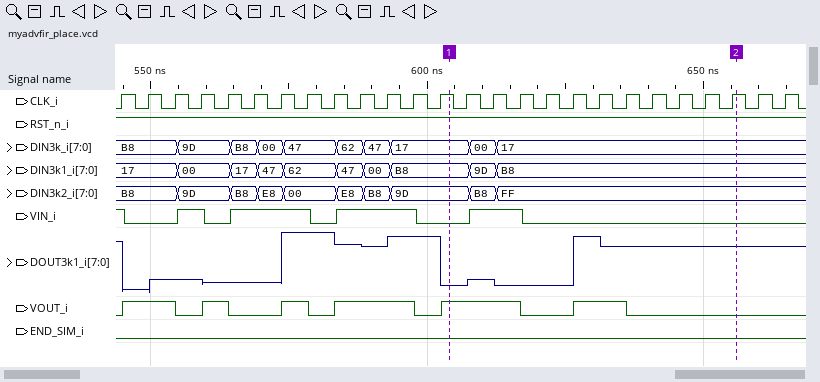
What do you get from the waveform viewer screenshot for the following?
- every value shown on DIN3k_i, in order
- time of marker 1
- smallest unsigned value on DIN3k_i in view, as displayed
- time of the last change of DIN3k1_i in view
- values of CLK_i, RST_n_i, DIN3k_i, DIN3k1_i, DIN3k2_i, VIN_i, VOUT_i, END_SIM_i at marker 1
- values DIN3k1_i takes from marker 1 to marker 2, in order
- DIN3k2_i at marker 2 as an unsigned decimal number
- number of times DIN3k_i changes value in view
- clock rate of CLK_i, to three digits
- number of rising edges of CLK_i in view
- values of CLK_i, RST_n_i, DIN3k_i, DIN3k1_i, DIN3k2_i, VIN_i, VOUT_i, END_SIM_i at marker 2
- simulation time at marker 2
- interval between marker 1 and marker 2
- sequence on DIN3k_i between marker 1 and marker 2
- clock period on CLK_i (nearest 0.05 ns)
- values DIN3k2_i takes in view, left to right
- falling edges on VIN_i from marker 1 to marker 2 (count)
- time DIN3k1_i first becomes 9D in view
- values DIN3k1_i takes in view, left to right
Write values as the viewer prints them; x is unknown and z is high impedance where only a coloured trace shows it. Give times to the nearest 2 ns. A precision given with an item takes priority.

B8, 9D, B8, 00, 47, 62, 47, 17, 00, 17
604 ns
00
612 ns
CLK_i=1, RST_n_i=1, DIN3k_i=17, DIN3k1_i=B8, DIN3k2_i=9D, VIN_i=0, VOUT_i=1, END_SIM_i=0
B8, 9D, B8
255
9
208 MHz
26
CLK_i=1, RST_n_i=1, DIN3k_i=17, DIN3k1_i=B8, DIN3k2_i=FF, VIN_i=0, VOUT_i=0, END_SIM_i=0
656 ns
52 ns
17, 00, 17
4.8 ns
B8, 9D, B8, E8, 00, E8, B8, 9D, B8, FF
1
608 ns
17, 00, 17, 47, 62, 47, 00, B8, 9D, B8
